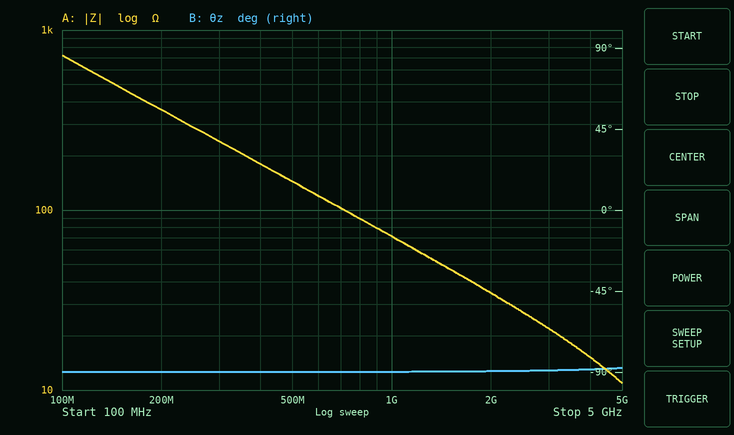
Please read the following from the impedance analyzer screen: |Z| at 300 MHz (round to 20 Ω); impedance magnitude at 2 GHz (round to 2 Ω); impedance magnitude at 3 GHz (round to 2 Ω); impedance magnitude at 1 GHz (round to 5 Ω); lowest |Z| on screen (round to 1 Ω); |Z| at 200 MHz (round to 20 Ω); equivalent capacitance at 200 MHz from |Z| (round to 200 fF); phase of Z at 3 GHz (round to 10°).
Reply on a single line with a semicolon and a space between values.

240 Ω; 34 Ω; 22 Ω; 70 Ω; 11 Ω; 360 Ω; 2.2 pF; -90°
